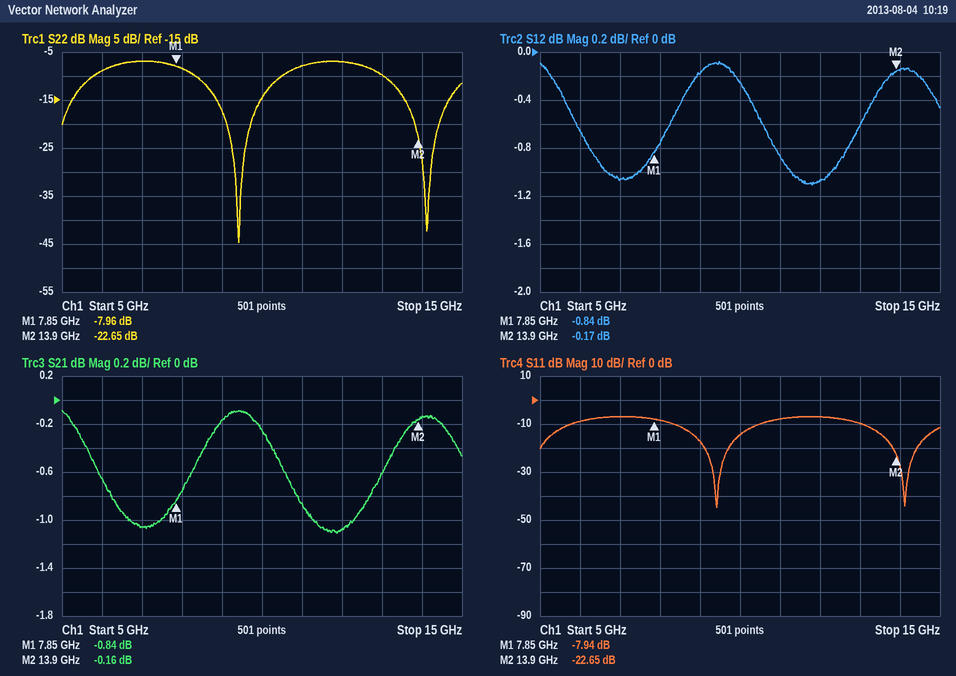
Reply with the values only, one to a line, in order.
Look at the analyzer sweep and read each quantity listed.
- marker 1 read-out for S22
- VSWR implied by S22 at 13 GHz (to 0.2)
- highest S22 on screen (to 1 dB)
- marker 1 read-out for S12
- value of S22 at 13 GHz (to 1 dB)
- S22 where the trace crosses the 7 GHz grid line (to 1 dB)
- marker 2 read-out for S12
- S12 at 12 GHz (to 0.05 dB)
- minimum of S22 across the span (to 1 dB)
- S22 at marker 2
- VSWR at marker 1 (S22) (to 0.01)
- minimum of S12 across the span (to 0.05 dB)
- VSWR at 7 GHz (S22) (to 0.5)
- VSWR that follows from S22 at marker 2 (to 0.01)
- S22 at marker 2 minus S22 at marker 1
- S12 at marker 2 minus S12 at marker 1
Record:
-7.96 dB
2.0
-7 dB
-0.84 dB
-10 dB
-7 dB
-0.17 dB
-1.05 dB
-45 dB
-22.65 dB
2.33
-1.10 dB
2.5
1.16
-14.69 dB
0.67 dB
